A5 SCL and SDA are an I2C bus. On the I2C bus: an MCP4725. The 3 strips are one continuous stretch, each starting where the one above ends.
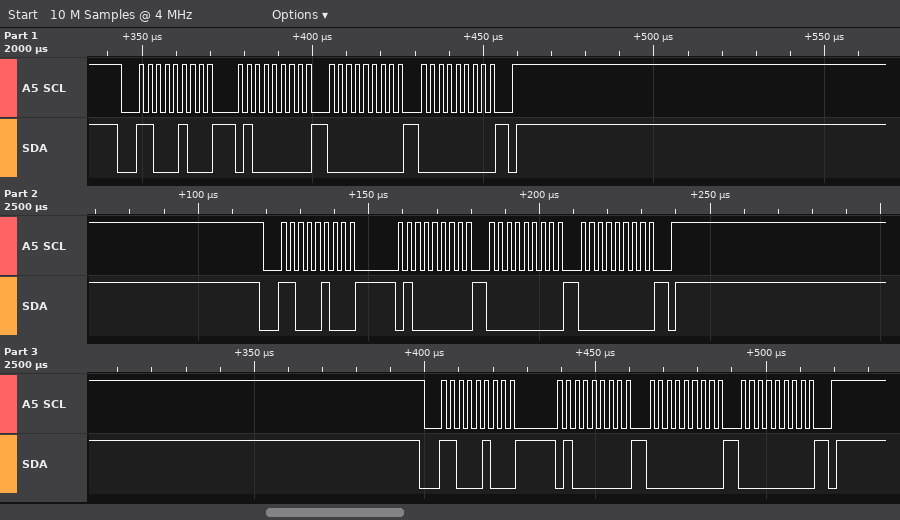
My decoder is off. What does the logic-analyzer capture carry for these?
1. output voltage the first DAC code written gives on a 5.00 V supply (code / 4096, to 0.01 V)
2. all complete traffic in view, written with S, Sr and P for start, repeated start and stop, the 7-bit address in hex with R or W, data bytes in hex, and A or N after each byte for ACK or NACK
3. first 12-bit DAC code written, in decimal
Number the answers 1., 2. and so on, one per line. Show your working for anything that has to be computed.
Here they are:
1. 0 / 4096 x 5.00 V = 0.00 V
2. S 62W A 40 A 00 A 00 A P S 62W A 40 A 00 A 00 A P S 62W A 40 A 00 A 00 A P
3. 0
